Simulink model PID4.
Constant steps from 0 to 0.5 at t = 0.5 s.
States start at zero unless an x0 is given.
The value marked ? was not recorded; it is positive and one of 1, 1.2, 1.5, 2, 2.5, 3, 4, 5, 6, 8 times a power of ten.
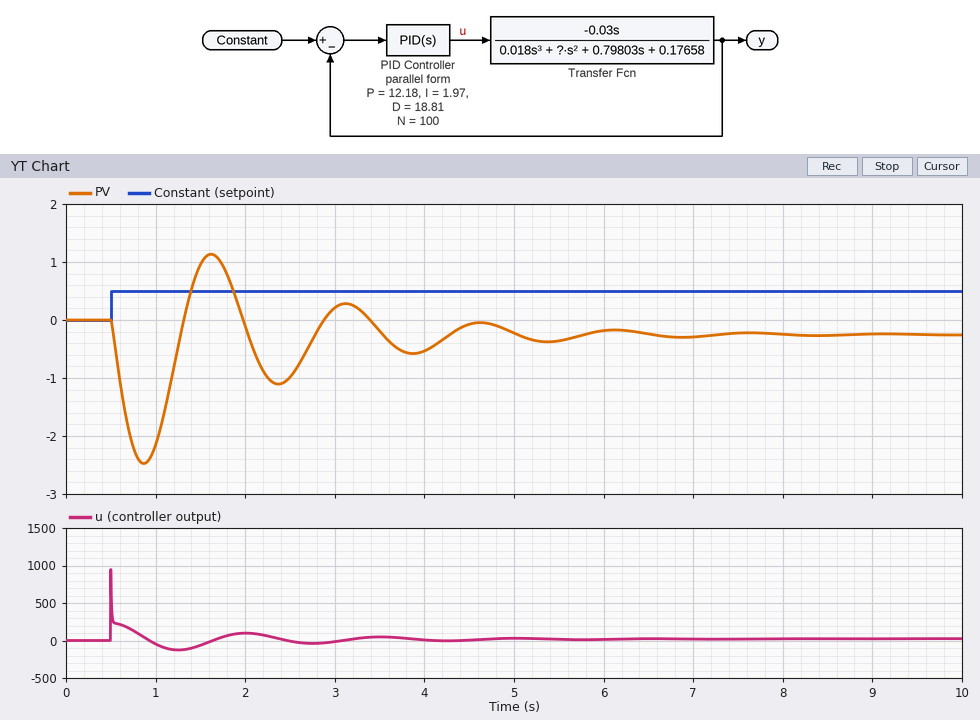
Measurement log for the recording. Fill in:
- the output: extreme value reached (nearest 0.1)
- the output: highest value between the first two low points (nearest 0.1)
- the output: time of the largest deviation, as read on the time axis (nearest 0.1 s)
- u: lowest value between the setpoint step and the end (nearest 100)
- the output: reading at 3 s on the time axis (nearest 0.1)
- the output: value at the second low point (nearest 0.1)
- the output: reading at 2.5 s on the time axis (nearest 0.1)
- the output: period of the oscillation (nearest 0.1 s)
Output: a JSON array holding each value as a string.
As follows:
["-2.5", "1.1", "0.9 s", "-100", "0.2", "-1.1", "-1.0", "1.5 s"]
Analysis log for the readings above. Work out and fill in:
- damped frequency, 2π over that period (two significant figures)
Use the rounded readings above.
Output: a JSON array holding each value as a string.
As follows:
["4.2 rad/s"]
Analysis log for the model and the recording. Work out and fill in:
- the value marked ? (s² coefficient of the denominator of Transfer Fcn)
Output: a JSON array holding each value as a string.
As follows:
["0.6"]
